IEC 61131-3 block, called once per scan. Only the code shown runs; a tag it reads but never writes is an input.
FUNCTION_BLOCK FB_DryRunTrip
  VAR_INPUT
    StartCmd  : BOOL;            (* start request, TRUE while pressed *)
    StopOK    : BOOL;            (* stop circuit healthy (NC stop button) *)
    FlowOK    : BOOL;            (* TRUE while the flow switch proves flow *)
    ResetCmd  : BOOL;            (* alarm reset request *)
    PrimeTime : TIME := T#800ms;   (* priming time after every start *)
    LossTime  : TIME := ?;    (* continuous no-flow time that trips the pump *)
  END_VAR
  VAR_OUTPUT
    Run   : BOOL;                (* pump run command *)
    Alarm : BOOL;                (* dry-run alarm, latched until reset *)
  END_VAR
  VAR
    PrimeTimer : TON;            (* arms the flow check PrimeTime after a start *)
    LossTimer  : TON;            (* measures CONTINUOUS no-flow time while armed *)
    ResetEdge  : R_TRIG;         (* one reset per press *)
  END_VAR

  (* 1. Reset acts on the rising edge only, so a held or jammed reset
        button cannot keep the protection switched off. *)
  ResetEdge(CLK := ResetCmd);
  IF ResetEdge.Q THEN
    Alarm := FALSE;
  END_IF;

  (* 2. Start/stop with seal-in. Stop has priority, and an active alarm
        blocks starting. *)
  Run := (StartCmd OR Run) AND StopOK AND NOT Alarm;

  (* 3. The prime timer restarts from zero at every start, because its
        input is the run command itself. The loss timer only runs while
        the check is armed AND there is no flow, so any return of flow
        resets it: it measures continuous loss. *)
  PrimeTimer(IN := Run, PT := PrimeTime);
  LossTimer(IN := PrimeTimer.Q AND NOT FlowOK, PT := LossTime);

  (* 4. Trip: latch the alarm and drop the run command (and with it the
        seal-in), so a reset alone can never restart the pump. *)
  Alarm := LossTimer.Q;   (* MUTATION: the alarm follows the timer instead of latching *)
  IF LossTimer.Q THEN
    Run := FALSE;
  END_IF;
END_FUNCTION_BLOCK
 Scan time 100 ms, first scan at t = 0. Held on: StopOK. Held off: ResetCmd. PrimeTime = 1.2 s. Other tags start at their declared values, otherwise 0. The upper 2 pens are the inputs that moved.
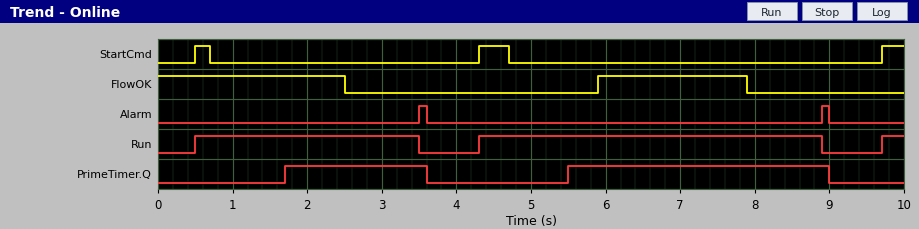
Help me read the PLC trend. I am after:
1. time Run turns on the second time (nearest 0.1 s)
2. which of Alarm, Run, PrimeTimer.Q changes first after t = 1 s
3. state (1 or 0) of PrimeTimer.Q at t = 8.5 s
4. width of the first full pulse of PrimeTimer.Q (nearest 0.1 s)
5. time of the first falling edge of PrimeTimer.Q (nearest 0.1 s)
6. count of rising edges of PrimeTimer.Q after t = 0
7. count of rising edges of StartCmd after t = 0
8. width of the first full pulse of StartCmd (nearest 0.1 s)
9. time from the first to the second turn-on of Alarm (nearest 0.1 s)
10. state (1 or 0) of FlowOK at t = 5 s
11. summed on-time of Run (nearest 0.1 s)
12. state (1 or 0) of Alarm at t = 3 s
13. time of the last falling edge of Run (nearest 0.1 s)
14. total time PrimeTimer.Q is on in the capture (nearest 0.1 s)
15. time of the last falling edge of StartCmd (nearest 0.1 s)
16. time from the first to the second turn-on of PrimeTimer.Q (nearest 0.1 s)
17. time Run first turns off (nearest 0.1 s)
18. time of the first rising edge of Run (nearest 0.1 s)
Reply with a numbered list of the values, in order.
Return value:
1. 4.3 s
2. PrimeTimer.Q
3. 1
4. 1.9 s
5. 3.6 s
6. 2
7. 3
8. 0.2 s
9. 5.4 s
10. 0
11. 7.9 s
12. 0
13. 8.9 s
14. 5.4 s
15. 4.7 s
16. 3.8 s
17. 3.5 s
18. 0.5 s
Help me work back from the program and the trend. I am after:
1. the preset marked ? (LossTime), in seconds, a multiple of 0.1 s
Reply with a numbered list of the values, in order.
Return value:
1. 1.0 s
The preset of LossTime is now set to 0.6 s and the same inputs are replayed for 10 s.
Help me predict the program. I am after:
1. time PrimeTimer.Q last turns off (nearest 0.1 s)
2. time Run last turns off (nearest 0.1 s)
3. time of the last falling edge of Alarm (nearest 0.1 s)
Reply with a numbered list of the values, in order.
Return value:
1. 8.6 s
2. 8.5 s
3. 8.6 s
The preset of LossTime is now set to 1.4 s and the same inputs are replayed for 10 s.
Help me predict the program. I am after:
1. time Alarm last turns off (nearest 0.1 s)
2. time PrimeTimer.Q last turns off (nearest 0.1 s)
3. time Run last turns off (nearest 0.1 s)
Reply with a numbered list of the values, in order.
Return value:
1. 9.4 s
2. 9.4 s
3. 9.3 s
